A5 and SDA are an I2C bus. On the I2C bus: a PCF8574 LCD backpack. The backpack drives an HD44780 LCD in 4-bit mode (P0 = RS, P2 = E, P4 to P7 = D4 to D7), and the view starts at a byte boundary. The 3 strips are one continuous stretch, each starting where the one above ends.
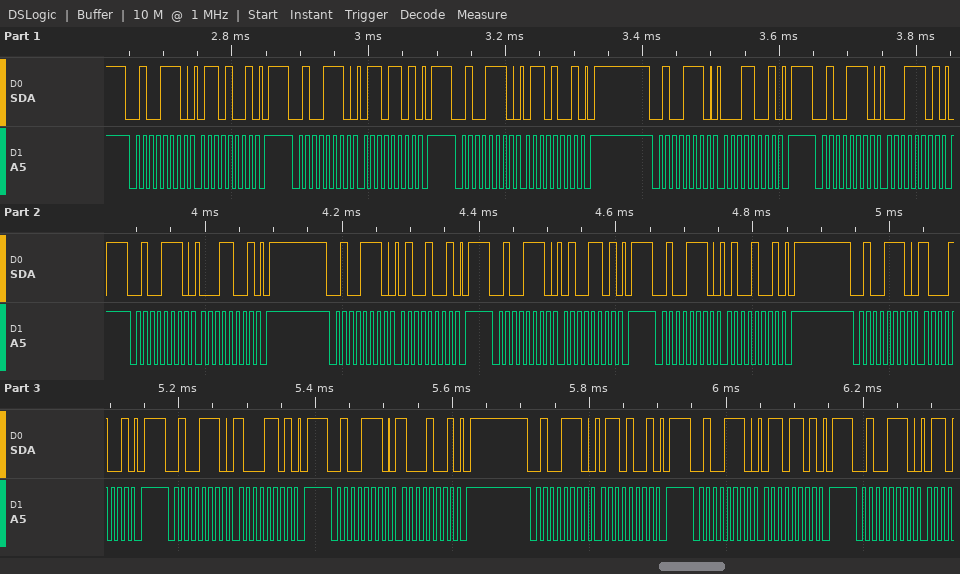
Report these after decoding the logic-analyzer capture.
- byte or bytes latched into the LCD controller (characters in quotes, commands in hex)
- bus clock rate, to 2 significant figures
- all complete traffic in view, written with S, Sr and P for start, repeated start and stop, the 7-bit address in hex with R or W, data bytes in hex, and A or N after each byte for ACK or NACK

'a' 'H'
100 kHz
S 27W A 69 A P S 27W A 6D A P S 27W A 69 A P S 27W A 19 A P S 27W A 1D A P S 27W A 19 A P S 27W A 49 A P S 27W A 4D A P S 27W A 49 A P S 27W A 89 A P S 27W A 8D A P S 27W A 89 A P S 27W A 69 A P S 27W A 6D A P S 27W A
